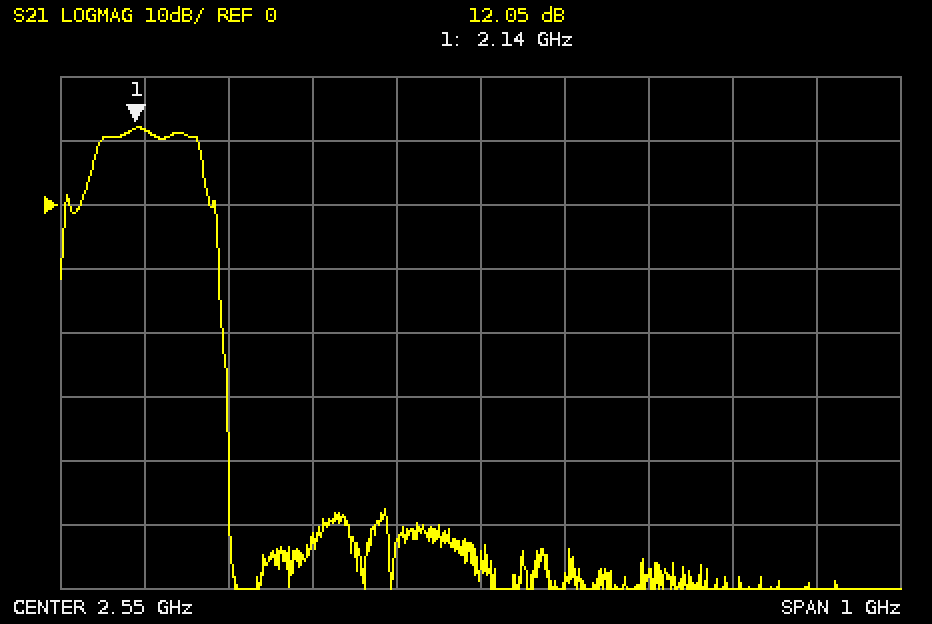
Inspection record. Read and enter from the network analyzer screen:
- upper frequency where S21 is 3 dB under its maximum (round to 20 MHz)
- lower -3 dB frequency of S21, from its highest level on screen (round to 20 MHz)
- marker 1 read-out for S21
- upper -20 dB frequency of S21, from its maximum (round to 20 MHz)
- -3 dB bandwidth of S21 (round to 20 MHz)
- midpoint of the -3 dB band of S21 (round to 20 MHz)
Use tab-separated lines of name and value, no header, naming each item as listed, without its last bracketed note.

upper frequency where S21 is 3 dB under its maximum	2.22 GHz
lower -3 dB frequency of S21, from its highest level on screen	2.10 GHz
marker 1 read-out for S21	12.05 dB
upper -20 dB frequency of S21, from its maximum	2.24 GHz
-3 dB bandwidth of S21	120 MHz
midpoint of the -3 dB band of S21	2.16 GHz
